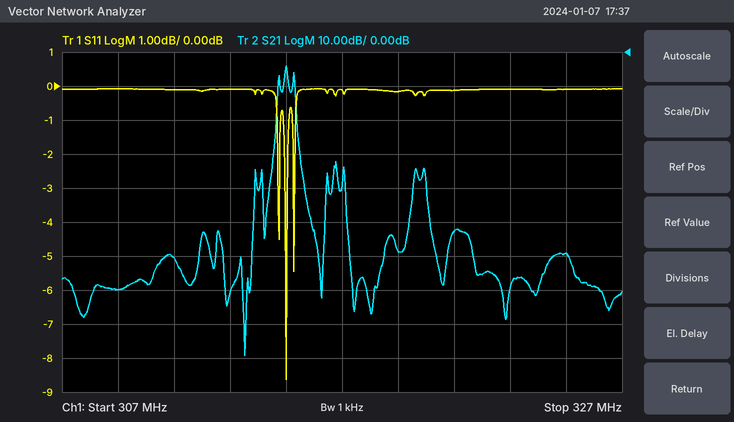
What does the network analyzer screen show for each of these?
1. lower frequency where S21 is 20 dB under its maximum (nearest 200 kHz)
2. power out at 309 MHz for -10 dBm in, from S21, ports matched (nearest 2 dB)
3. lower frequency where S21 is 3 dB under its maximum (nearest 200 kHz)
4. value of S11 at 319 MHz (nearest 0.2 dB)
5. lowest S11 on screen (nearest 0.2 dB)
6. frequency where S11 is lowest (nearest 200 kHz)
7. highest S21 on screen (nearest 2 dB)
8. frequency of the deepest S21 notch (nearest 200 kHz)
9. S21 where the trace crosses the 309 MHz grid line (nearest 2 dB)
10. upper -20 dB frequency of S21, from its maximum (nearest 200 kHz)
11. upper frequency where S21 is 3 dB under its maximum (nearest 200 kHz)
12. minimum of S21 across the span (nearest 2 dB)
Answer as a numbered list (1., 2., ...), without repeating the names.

1. 314.6 MHz
2. -80 dBm
3. 315.0 MHz
4. -0.2 dB
5. -8.6 dB
6. 315.0 MHz
7. -4 dB
8. 313.6 MHz
9. -70 dB
10. 315.4 MHz
11. 315.0 MHz
12. -90 dB
